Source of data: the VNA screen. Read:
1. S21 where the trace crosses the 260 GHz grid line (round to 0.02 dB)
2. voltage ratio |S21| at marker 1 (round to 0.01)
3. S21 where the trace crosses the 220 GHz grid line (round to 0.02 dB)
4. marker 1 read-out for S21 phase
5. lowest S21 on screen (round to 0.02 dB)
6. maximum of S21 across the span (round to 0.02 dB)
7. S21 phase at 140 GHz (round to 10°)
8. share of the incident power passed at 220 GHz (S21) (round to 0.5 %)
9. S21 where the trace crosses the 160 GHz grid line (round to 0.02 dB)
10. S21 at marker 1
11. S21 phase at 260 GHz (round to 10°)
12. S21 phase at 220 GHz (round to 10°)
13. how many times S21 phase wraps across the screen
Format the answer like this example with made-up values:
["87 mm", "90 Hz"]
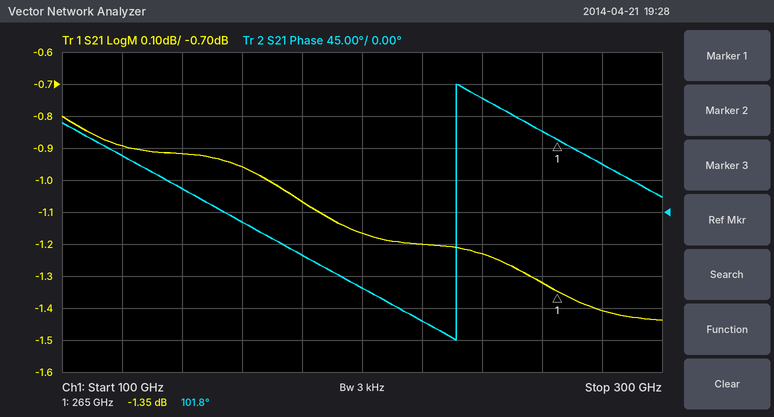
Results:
["-1.32 dB", "0.86", "-1.20 dB", "101.8°", "-1.44 dB", "-0.80 dB", "30°", "76.0 %", "-0.96 dB", "-1.35 dB", "110°", "-150°", "1"]
